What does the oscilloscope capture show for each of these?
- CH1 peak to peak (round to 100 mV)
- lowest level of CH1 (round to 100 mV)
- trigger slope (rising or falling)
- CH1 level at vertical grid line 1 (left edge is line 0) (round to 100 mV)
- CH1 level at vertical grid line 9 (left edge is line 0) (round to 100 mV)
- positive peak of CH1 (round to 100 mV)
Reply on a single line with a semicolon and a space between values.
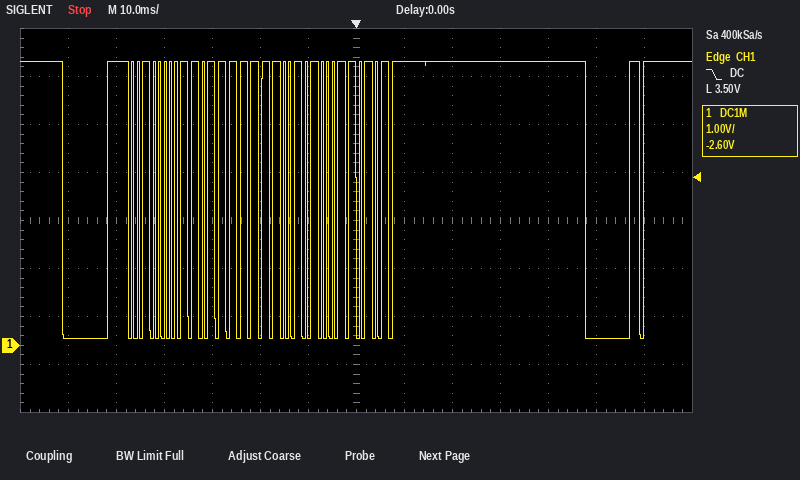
5.8 V; 100 mV; falling; 100 mV; 5.9 V; 5.9 V
